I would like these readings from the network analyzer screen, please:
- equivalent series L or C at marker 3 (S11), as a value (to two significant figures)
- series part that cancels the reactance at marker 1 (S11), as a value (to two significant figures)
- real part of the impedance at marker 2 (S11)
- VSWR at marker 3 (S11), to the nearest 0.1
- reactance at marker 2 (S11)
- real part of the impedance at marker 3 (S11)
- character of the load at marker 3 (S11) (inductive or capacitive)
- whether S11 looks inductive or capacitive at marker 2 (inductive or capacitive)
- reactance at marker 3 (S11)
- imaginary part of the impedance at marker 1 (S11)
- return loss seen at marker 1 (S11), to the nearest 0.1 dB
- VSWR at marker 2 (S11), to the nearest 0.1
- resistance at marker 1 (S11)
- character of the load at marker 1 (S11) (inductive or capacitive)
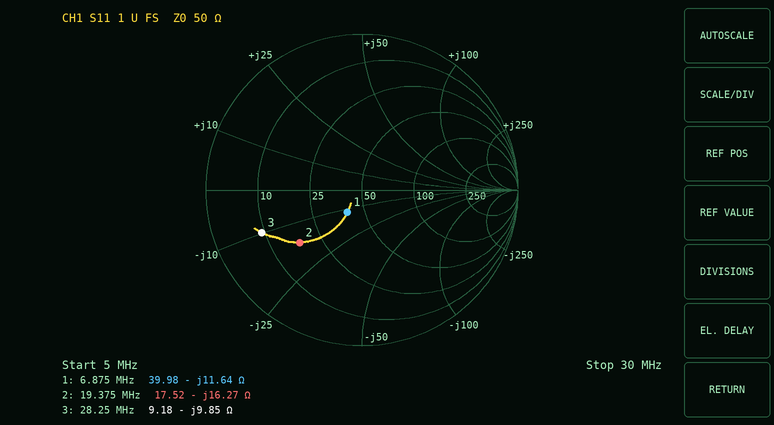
570 pF
270 nH
17.52 Ω
5.7
-16.27 Ω
9.18 Ω
capacitive
capacitive
-9.85 Ω
-11.64 Ω
15.4 dB
3.2
39.98 Ω
capacitive
